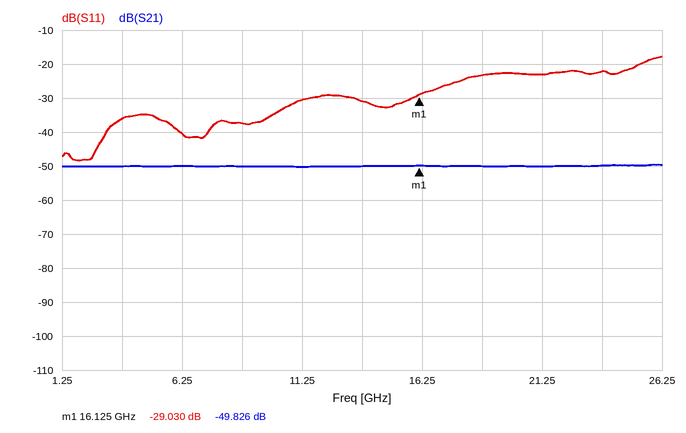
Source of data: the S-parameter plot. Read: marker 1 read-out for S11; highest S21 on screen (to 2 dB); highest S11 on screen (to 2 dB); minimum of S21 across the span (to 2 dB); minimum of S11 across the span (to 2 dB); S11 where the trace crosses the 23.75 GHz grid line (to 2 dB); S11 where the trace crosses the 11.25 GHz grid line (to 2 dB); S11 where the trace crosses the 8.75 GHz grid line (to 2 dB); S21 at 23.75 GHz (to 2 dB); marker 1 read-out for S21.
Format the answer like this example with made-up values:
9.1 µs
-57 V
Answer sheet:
-29.030 dB
-50 dB
-18 dB
-50 dB
-48 dB
-22 dB
-30 dB
-38 dB
-50 dB
-49.826 dB
